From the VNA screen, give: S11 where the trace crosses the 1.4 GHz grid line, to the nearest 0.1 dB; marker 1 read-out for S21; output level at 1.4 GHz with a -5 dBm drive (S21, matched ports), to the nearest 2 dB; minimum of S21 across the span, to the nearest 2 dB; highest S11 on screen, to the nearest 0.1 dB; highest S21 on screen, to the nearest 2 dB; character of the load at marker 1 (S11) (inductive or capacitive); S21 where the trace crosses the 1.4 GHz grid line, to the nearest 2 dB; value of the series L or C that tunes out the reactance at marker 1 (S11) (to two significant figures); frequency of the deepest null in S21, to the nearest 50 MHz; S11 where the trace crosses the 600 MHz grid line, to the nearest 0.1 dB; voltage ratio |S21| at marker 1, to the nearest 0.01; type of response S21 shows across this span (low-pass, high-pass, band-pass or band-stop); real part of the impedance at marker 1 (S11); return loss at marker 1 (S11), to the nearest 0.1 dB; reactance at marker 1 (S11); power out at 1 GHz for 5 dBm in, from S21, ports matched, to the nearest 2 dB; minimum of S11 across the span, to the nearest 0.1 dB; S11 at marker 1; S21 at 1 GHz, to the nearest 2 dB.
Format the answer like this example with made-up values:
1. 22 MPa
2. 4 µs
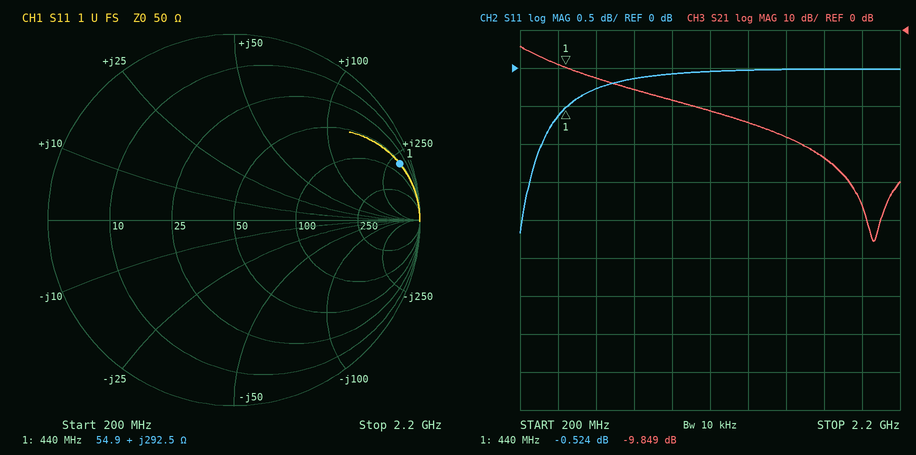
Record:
1. 0.0 dB
2. -9.849 dB
3. -30 dBm
4. -56 dB
5. 0.0 dB
6. -4 dB
7. inductive
8. -24 dB
9. 1.2 pF
10. 2.05 GHz
11. -0.3 dB
12. 0.32
13. low-pass
14. 54.9 Ω
15. 0.5 dB
16. +292.5 Ω
17. -14 dBm
18. -2.2 dB
19. -0.524 dB
20. -18 dB
